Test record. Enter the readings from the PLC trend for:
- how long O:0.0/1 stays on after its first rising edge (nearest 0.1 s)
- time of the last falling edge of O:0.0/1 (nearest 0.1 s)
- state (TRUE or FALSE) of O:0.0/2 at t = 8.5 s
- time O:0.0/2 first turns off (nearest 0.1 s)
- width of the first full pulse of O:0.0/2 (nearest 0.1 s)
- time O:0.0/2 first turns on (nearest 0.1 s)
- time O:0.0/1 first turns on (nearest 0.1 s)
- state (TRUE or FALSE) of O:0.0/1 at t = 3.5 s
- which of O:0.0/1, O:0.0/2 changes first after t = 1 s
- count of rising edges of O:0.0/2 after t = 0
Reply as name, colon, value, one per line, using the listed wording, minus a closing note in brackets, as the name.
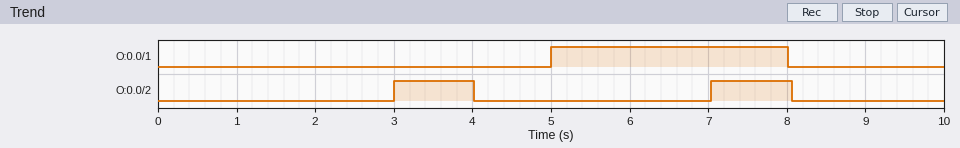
how long O:0.0/1 stays on after its first rising edge: 3.0 s
time of the last falling edge of O:0.0/1: 8.0 s
state (TRUE or FALSE) of O:0.0/2 at t = 8.5 s: FALSE
time O:0.0/2 first turns off: 4.0 s
width of the first full pulse of O:0.0/2: 1.0 s
time O:0.0/2 first turns on: 3.0 s
time O:0.0/1 first turns on: 5.0 s
state (TRUE or FALSE) of O:0.0/1 at t = 3.5 s: FALSE
which of O:0.0/1, O:0.0/2 changes first after t = 1 s: O:0.0/2
count of rising edges of O:0.0/2 after t = 0: 2
